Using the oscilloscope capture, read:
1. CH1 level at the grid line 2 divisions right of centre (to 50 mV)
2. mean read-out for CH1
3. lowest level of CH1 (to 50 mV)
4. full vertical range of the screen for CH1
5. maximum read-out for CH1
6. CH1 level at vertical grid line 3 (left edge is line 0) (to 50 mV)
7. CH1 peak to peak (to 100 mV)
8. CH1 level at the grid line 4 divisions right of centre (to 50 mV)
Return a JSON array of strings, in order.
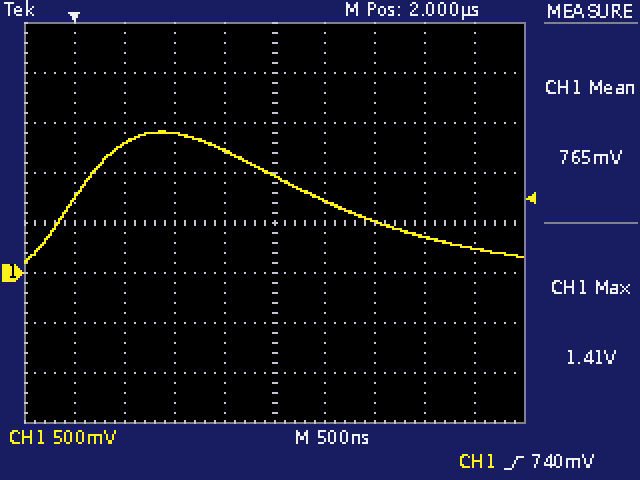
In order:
["500 mV", "765 mV", "100 mV", "4 V", "1.41 V", "1.40 V", "1.30 V", "250 mV"]
